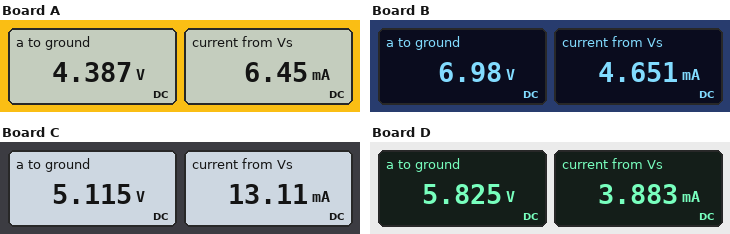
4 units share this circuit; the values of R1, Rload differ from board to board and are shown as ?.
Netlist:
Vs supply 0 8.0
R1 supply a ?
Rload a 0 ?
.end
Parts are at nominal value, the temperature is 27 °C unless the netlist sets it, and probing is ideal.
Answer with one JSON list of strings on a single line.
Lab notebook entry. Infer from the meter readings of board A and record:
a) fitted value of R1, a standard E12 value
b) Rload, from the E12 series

["560 Ω", "680 Ω"]
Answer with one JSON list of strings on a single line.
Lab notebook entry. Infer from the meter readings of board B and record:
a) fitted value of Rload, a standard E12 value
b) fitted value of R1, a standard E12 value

["1.5 kΩ", "220 Ω"]
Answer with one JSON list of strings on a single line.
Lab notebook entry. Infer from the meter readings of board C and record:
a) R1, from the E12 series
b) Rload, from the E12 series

["220 Ω", "390 Ω"]
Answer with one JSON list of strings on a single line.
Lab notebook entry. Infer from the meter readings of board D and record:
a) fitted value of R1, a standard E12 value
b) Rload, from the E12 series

["560 Ω", "1.5 kΩ"]
